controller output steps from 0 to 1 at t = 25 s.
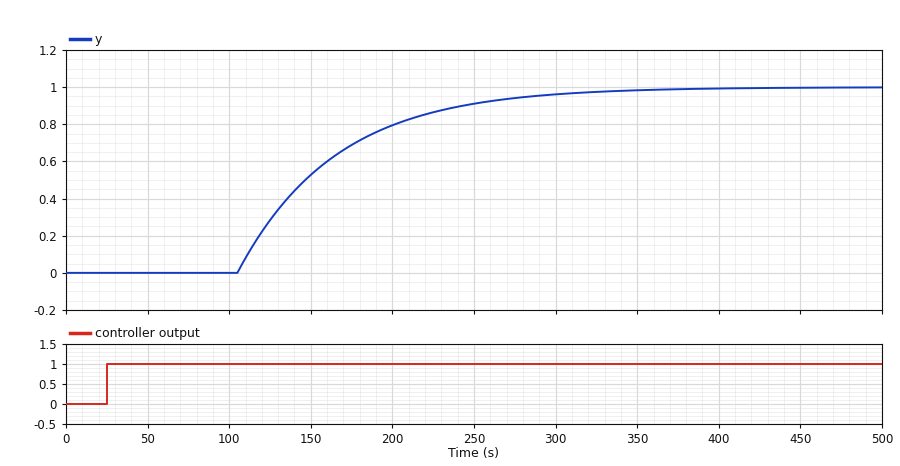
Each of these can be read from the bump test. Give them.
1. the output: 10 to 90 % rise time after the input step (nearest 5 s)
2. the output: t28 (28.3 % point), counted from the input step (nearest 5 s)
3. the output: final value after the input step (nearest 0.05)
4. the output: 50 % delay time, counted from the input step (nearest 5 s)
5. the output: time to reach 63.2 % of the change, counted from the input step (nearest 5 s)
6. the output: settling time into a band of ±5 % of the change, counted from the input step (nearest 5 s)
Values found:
130 s
100 s
1.00
120 s
140 s
260 s
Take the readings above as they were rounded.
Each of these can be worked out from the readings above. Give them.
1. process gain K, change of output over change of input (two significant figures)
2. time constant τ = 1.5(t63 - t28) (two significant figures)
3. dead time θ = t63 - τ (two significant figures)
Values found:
1.0
60 s
80 s
